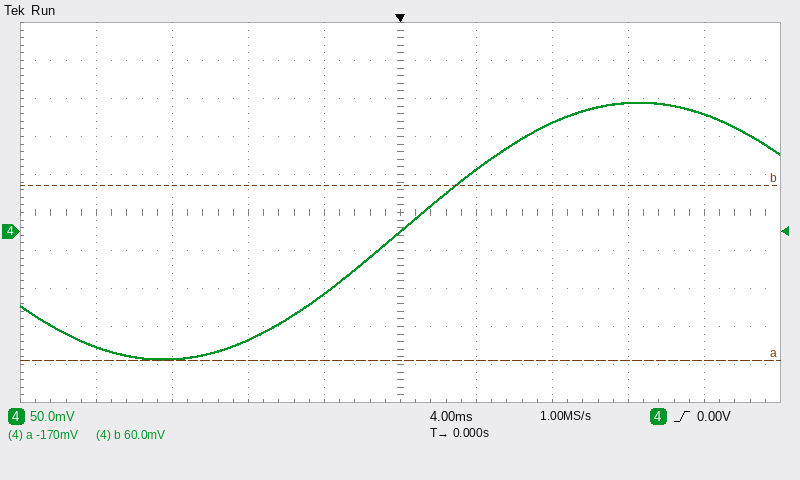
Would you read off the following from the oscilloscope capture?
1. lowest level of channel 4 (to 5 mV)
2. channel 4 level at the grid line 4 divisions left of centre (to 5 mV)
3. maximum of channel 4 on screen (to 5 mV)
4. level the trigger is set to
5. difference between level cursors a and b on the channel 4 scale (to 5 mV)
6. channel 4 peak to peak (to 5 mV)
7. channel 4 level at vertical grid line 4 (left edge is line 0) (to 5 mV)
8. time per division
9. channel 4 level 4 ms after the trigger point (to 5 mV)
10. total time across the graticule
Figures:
-170 mV
-150 mV
170 mV
0.00 V
230 mV
340 mV
-80 mV
4 ms
80 mV
40 ms
